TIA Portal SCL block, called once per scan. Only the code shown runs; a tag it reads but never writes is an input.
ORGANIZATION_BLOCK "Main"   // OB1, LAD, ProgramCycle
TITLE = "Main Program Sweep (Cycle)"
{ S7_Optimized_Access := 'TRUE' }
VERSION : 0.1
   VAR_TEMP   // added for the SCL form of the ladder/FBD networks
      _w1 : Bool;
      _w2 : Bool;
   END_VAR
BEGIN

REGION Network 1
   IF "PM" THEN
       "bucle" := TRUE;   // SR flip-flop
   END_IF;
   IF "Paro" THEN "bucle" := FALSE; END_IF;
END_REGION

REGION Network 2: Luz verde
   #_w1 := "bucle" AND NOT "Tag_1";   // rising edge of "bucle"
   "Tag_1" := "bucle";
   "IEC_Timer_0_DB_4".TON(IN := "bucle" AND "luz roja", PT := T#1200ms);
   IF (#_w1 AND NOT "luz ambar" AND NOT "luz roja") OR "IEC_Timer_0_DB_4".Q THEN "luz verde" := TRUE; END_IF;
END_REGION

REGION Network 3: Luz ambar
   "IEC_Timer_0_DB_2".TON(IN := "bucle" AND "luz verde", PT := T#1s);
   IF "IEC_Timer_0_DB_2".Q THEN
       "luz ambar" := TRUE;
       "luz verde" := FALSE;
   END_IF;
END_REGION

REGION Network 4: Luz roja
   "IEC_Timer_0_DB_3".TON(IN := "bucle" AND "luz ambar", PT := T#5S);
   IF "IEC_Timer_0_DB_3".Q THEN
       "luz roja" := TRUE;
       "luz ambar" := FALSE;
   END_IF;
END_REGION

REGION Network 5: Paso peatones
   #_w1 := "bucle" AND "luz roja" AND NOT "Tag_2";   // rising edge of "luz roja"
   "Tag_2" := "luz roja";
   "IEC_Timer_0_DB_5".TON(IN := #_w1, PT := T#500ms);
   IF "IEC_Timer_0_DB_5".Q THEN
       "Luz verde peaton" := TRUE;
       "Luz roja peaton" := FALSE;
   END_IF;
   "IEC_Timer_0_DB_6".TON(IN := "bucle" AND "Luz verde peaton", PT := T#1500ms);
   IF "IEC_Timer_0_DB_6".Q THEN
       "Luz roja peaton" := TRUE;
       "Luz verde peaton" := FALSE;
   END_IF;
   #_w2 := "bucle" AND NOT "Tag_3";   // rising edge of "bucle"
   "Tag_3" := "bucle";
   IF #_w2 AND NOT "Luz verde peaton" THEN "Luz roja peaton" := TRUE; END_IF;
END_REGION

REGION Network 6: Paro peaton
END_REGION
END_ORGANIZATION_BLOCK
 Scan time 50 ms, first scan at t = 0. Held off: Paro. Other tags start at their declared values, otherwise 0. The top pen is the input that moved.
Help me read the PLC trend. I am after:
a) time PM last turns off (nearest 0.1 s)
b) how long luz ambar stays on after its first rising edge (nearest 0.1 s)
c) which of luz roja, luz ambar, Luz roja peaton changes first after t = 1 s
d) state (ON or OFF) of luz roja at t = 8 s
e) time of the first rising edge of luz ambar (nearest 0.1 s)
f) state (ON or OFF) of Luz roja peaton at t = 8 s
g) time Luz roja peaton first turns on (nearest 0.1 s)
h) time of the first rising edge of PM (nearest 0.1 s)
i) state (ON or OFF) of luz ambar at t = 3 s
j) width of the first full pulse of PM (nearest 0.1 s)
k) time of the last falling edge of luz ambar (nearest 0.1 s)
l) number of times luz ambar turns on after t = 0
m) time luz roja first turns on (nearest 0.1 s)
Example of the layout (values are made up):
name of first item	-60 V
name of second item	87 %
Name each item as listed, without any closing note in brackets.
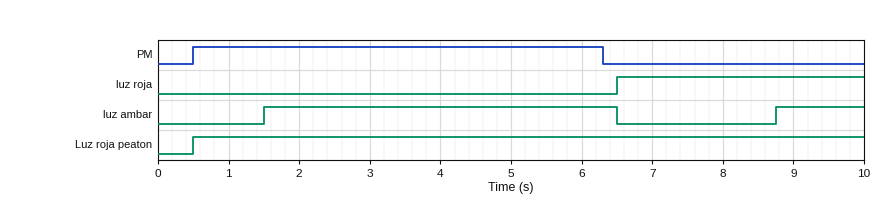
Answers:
time PM last turns off	6.3 s
how long luz ambar stays on after its first rising edge	5.0 s
which of luz roja, luz ambar, Luz roja peaton changes first after t = 1 s	luz ambar
state (ON or OFF) of luz roja at t = 8 s	ON
time of the first rising edge of luz ambar	1.5 s
state (ON or OFF) of Luz roja peaton at t = 8 s	ON
time Luz roja peaton first turns on	0.5 s
time of the first rising edge of PM	0.5 s
state (ON or OFF) of luz ambar at t = 3 s	ON
width of the first full pulse of PM	5.8 s
time of the last falling edge of luz ambar	6.5 s
number of times luz ambar turns on after t = 0	2
time luz roja first turns on	6.5 s
